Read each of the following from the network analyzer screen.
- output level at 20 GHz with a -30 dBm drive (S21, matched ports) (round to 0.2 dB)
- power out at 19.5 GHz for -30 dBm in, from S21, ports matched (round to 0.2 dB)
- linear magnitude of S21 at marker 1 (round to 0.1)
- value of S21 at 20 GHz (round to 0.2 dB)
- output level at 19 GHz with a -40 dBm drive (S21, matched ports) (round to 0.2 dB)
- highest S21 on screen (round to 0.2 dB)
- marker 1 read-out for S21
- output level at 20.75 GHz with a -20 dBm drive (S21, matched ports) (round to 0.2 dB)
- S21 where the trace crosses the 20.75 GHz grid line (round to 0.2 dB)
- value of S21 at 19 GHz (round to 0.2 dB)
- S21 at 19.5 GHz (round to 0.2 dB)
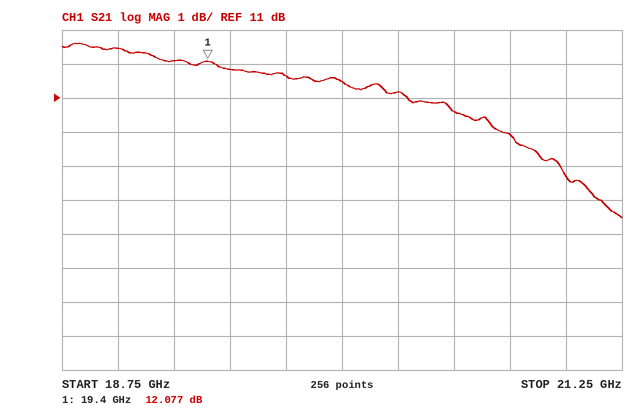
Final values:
-18.6 dBm
-18.2 dBm
4.0
11.4 dB
-27.6 dBm
12.6 dB
12.077 dB
-10.0 dBm
10.0 dB
12.4 dB
11.8 dB
